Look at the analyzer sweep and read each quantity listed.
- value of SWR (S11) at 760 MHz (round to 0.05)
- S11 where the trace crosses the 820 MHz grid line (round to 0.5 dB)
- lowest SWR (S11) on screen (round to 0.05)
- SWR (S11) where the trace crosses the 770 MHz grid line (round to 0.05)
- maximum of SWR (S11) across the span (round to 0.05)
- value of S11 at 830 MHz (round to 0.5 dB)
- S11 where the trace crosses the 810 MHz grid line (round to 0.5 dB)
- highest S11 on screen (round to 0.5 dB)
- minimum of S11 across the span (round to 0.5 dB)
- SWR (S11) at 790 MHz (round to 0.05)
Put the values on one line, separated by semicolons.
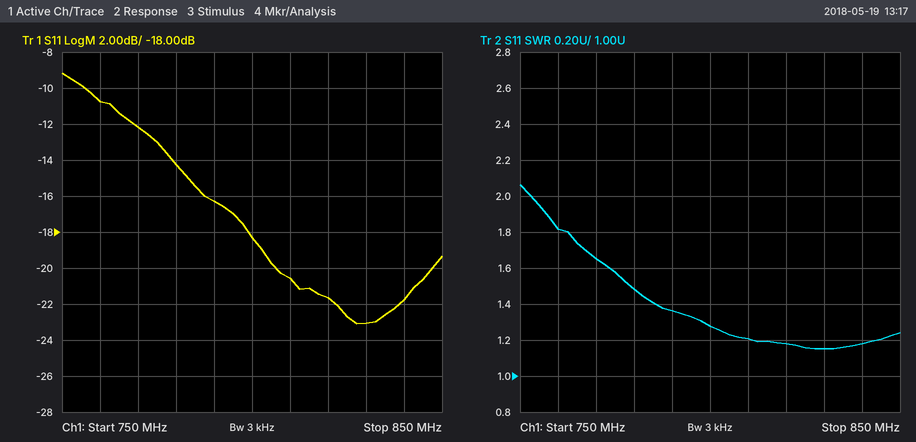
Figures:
1.80; -21.5 dB; 1.15; 1.65; 2.05; -23.0 dB; -20.5 dB; -9.0 dB; -23.0 dB; 1.35
